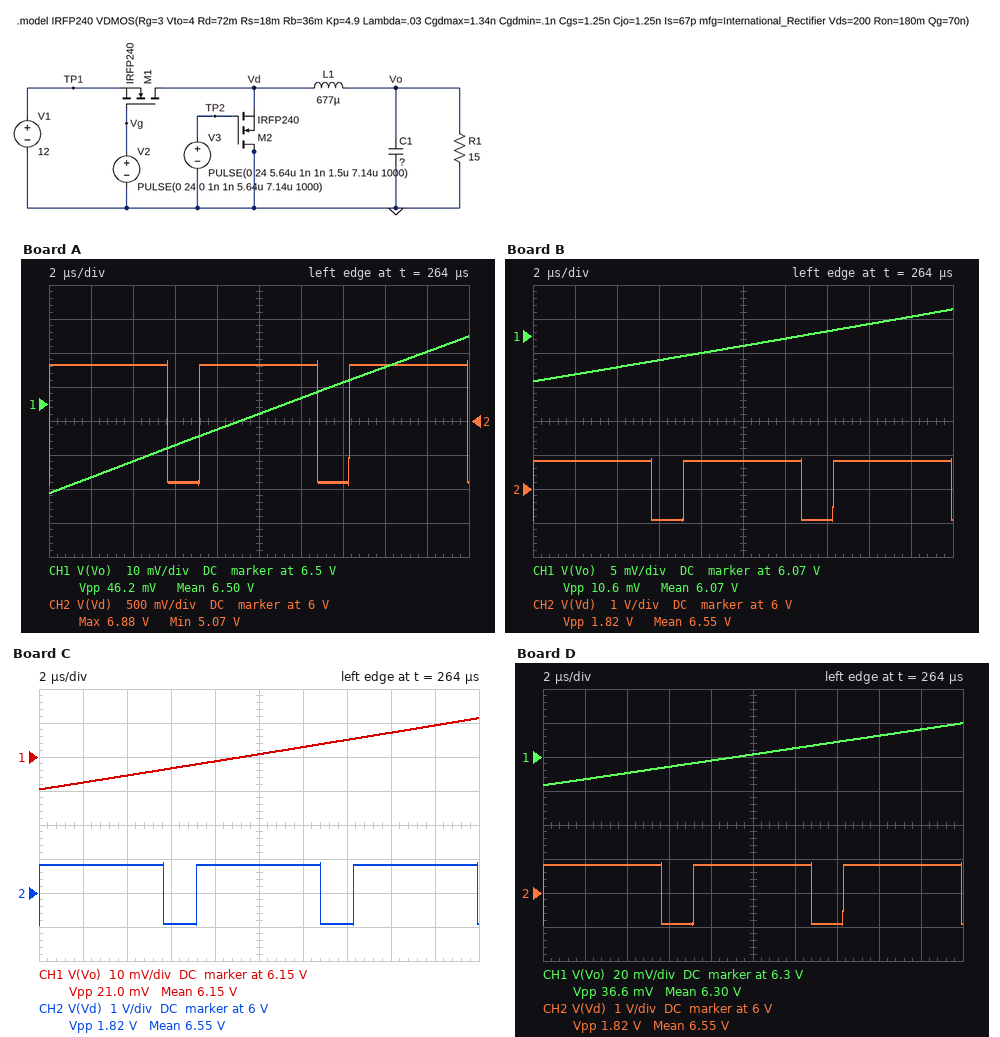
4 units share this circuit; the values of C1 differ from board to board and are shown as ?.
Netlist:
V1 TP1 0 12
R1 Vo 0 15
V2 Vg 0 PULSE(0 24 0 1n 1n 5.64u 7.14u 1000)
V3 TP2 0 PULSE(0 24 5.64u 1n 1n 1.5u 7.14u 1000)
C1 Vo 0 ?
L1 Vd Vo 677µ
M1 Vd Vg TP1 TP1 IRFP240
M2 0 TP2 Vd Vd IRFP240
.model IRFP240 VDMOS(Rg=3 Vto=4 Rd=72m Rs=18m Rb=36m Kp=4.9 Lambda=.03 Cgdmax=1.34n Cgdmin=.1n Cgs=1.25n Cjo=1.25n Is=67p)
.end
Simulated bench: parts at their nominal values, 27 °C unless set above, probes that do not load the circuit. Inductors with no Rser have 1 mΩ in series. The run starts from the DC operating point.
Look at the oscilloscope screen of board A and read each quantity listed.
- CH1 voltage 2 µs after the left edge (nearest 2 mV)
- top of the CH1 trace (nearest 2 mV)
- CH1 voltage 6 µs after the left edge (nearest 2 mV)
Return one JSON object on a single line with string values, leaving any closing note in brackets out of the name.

{"CH1 voltage 2 µs after the left edge": "6.478 V", "top of the CH1 trace": "6.520 V", "CH1 voltage 6 µs after the left edge": "6.488 V"}
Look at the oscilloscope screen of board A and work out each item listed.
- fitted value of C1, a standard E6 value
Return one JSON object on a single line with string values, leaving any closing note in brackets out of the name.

{"fitted value of C1, a standard E6 value": "33 µF"}
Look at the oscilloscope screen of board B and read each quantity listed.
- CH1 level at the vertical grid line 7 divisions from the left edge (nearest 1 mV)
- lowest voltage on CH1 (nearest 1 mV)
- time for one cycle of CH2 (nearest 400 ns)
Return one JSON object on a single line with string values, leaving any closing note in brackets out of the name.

{"CH1 level at the vertical grid line 7 divisions from the left edge": "6.071 V", "lowest voltage on CH1": "6.063 V", "time for one cycle of CH2": "7.2 µs"}
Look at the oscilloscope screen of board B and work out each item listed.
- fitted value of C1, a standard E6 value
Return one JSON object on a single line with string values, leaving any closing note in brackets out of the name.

{"fitted value of C1, a standard E6 value": "330 µF"}
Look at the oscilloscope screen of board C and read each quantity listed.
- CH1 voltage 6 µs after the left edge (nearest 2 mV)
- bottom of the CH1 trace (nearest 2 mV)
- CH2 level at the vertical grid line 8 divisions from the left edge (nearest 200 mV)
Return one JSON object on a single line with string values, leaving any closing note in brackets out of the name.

{"CH1 voltage 6 µs after the left edge": "6.146 V", "bottom of the CH1 trace": "6.140 V", "CH2 level at the vertical grid line 8 divisions from the left edge": "6.8 V"}
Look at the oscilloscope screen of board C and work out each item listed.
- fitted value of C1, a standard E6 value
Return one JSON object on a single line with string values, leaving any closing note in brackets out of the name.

{"fitted value of C1, a standard E6 value": "150 µF"}
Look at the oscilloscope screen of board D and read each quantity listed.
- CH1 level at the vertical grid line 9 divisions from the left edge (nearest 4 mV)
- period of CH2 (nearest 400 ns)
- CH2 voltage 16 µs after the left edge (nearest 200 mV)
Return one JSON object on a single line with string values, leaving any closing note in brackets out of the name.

{"CH1 level at the vertical grid line 9 divisions from the left edge": "6.316 V", "period of CH2": "7.2 µs", "CH2 voltage 16 µs after the left edge": "6.8 V"}
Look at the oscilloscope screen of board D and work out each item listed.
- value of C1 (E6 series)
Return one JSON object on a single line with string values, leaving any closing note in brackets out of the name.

{"value of C1": "68 µF"}
